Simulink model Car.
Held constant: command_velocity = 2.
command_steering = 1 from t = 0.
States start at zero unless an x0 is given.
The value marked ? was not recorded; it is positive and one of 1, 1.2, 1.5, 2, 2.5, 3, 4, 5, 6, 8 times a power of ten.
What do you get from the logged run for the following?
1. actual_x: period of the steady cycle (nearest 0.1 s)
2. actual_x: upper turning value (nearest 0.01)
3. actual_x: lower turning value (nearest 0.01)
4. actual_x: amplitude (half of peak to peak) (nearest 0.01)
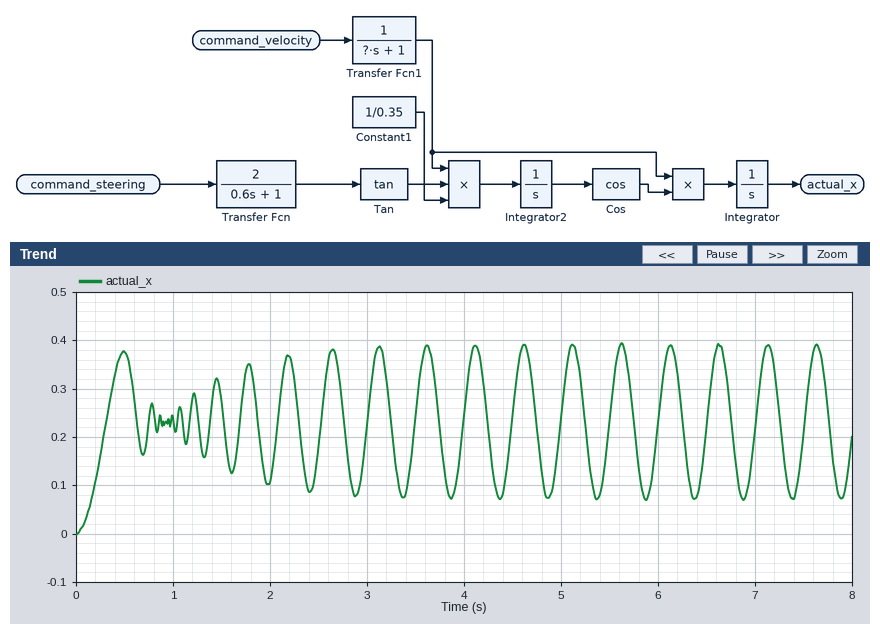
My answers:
0.5 s
0.39
0.07
0.16
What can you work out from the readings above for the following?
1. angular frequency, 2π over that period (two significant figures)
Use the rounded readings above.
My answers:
13 rad/s
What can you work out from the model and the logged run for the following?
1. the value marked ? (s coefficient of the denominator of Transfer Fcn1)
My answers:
0.3
